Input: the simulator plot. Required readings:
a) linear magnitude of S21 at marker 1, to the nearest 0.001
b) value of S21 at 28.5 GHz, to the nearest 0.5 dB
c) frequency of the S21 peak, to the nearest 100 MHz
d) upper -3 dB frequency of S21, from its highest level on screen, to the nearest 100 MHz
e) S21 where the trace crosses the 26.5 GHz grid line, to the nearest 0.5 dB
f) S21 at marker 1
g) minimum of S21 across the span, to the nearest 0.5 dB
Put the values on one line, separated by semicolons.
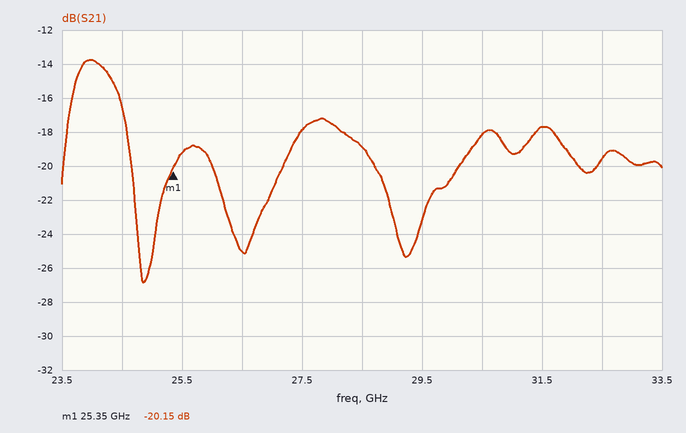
0.098; -19.0 dB; 24.0 GHz; 24.5 GHz; -25.0 dB; -20.15 dB; -27.0 dB
